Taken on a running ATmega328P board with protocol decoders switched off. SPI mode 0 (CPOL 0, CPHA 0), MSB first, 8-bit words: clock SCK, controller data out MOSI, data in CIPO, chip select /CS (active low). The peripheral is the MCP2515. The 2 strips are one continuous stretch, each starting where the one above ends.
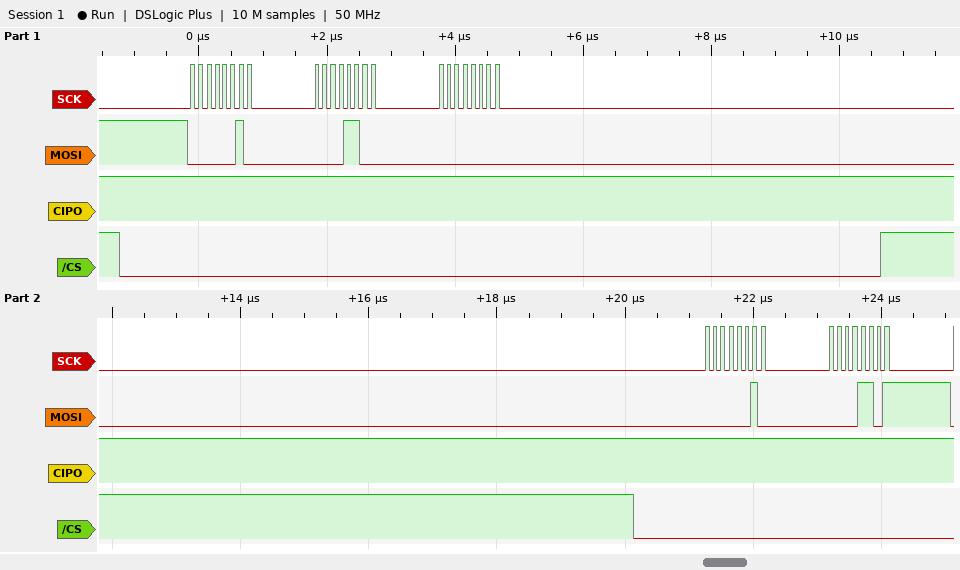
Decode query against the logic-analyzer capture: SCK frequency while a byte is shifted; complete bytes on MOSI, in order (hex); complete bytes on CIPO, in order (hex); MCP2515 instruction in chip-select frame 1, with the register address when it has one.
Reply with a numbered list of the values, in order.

1. 8 MHz
2. 02 0C 00 02 0D
3. FF FF FF FF FF
4. WRITE 0x0C
